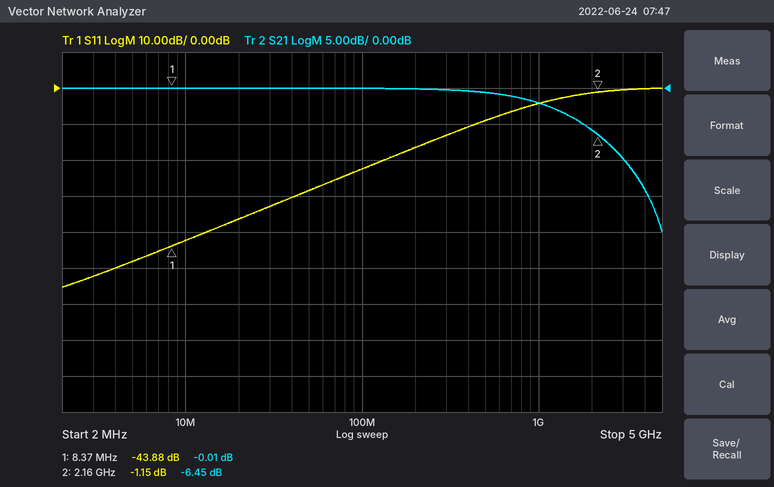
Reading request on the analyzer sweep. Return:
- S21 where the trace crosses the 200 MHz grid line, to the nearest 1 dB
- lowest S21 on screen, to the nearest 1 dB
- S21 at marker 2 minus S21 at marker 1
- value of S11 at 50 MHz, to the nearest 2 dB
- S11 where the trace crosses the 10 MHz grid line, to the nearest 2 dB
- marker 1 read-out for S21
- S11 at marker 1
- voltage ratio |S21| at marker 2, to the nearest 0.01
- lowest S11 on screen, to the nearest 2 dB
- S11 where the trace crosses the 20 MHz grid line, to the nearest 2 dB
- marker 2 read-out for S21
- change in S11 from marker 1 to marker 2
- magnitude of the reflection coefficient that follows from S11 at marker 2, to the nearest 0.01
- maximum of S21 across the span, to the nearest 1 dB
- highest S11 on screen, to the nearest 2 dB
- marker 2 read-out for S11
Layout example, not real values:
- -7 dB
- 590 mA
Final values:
- 0 dB
- -20 dB
- -6.44 dB
- -28 dB
- -42 dB
- -0.01 dB
- -43.88 dB
- 0.48
- -56 dB
- -36 dB
- -6.45 dB
- 42.73 dB
- 0.88
- 0 dB
- 0 dB
- -1.15 dB
